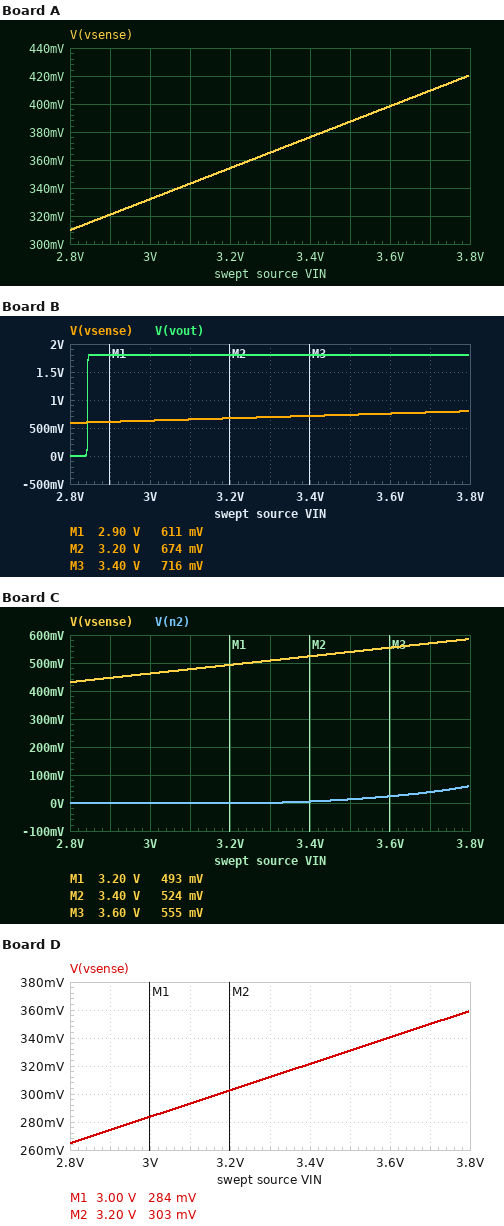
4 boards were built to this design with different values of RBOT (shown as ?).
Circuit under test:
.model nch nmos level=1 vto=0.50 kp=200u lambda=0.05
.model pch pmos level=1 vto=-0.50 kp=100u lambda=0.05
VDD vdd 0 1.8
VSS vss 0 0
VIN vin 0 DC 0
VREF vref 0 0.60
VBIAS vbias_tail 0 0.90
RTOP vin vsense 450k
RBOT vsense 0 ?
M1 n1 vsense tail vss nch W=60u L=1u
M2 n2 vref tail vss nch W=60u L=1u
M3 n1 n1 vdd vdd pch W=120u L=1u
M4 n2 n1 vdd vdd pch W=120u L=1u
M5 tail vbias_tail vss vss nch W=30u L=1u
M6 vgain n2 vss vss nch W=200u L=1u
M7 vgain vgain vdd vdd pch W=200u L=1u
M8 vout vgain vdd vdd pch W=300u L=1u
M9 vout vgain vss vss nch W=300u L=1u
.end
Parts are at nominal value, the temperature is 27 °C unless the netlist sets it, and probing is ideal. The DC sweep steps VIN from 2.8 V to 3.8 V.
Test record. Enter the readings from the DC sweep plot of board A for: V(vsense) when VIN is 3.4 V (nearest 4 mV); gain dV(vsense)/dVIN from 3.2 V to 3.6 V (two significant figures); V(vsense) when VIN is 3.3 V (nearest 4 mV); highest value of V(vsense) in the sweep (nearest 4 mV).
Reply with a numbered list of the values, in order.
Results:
1. 376 mV
2. 0.11 V/V
3. 364 mV
4. 420 mV
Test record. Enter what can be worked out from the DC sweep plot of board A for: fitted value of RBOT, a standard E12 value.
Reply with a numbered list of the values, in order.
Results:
1. 56 kΩ
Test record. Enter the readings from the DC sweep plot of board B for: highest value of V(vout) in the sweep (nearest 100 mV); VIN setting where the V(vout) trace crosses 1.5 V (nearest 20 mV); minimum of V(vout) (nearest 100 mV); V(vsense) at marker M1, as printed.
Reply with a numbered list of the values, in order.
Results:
1. 1.8 V
2. 2.84 V
3. 0 V
4. 611 mV
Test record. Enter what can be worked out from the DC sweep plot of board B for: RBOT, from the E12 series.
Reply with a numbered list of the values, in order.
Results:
1. 120 kΩ
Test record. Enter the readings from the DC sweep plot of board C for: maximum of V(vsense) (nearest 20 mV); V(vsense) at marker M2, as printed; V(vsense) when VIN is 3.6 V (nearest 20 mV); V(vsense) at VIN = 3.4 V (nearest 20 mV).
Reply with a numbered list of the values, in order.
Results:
1. 580 mV
2. 524 mV
3. 560 mV
4. 520 mV
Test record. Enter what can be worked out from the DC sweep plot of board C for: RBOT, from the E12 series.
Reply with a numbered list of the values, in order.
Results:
1. 82 kΩ
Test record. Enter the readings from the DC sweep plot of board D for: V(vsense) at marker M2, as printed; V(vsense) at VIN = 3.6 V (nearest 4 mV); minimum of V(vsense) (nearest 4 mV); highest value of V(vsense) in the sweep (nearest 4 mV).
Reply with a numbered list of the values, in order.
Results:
1. 303 mV
2. 340 mV
3. 264 mV
4. 360 mV
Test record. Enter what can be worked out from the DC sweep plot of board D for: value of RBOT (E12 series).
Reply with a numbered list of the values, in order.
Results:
1. 47 kΩ
